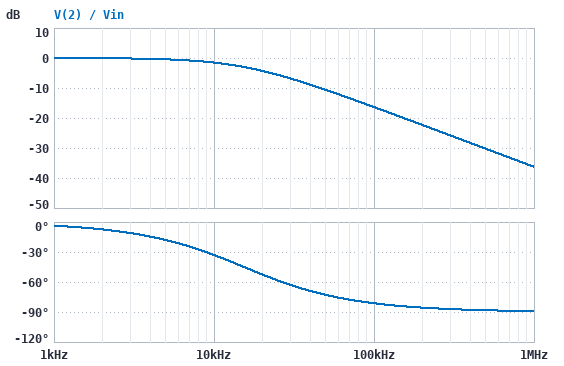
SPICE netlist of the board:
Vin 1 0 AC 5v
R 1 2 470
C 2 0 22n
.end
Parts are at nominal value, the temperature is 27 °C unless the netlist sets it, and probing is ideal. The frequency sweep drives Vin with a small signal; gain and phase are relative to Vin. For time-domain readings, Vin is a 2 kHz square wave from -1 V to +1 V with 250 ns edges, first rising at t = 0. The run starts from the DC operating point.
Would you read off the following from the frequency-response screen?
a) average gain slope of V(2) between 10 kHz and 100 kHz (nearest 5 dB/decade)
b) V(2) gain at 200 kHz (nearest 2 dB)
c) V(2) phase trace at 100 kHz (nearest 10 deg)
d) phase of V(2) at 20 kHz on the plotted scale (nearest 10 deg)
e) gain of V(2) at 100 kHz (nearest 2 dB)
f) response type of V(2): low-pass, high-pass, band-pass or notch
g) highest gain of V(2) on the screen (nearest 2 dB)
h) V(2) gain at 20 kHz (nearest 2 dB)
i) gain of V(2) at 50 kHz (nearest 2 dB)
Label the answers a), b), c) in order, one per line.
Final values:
a) -15 dB/decade
b) -22 dB
c) -80 deg
d) -50 deg
e) -16 dB
f) low-pass
g) 0 dB
h) -4 dB
i) -10 dB
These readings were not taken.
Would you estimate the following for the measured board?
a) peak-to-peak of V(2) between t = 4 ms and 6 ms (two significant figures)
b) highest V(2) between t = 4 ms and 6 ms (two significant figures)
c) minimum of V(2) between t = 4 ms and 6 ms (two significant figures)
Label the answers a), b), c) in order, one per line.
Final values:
a) 2.0 V
b) 1.0 V
c) -1.0 V
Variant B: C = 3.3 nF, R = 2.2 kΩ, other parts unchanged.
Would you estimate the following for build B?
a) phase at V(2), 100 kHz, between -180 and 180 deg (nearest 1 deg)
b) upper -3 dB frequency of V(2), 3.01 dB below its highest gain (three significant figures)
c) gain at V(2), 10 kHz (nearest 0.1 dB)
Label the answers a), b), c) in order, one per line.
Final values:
a) -78 deg
b) 21.9 kHz
c) -0.8 dB
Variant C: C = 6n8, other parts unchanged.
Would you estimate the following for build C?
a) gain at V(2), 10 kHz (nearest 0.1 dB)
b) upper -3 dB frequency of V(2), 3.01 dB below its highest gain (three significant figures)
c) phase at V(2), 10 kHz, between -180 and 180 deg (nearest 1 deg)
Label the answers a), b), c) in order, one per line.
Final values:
a) -0.2 dB
b) 49.8 kHz
c) -11 deg
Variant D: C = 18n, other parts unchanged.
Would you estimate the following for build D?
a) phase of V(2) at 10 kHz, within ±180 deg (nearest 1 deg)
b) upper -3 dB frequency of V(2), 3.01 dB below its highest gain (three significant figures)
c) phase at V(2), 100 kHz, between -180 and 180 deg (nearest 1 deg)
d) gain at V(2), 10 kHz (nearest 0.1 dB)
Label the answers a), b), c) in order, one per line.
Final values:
a) -28 deg
b) 18.8 kHz
c) -79 deg
d) -1.1 dB
